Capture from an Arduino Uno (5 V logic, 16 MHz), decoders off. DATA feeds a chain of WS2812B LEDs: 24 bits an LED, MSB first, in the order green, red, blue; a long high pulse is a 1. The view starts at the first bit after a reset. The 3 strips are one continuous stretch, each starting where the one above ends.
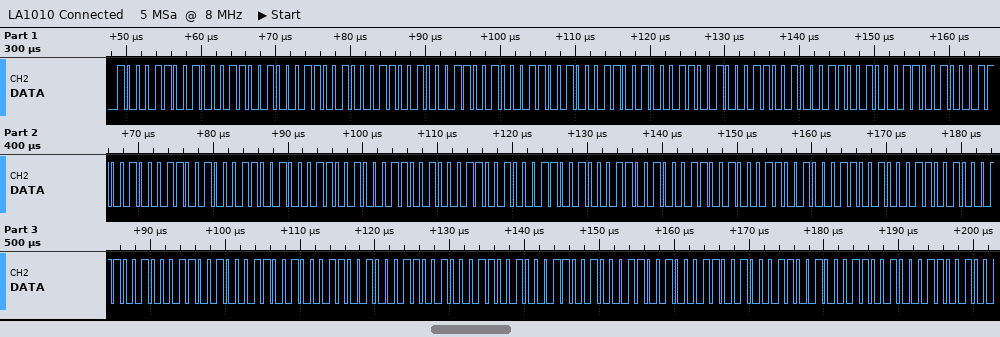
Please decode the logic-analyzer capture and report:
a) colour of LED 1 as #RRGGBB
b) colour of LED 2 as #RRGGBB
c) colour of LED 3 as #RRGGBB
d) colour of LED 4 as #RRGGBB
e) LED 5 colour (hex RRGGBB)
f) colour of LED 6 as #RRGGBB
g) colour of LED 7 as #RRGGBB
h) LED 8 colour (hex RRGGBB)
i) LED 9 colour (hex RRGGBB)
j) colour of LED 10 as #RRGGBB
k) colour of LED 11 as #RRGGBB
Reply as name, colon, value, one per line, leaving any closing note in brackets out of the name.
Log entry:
colour of LED 1 as #RRGGBB: #8C8C8C
colour of LED 2 as #RRGGBB: #8C8C8C
colour of LED 3 as #RRGGBB: #8C8C8C
colour of LED 4 as #RRGGBB: #8C8C8C
LED 5 colour: #8C8C8C
colour of LED 6 as #RRGGBB: #8C8C8C
colour of LED 7 as #RRGGBB: #8C8C8C
LED 8 colour: #8C8C8C
LED 9 colour: #8C8C8C
colour of LED 10 as #RRGGBB: #8C8C8C
colour of LED 11 as #RRGGBB: #8C8C8C
